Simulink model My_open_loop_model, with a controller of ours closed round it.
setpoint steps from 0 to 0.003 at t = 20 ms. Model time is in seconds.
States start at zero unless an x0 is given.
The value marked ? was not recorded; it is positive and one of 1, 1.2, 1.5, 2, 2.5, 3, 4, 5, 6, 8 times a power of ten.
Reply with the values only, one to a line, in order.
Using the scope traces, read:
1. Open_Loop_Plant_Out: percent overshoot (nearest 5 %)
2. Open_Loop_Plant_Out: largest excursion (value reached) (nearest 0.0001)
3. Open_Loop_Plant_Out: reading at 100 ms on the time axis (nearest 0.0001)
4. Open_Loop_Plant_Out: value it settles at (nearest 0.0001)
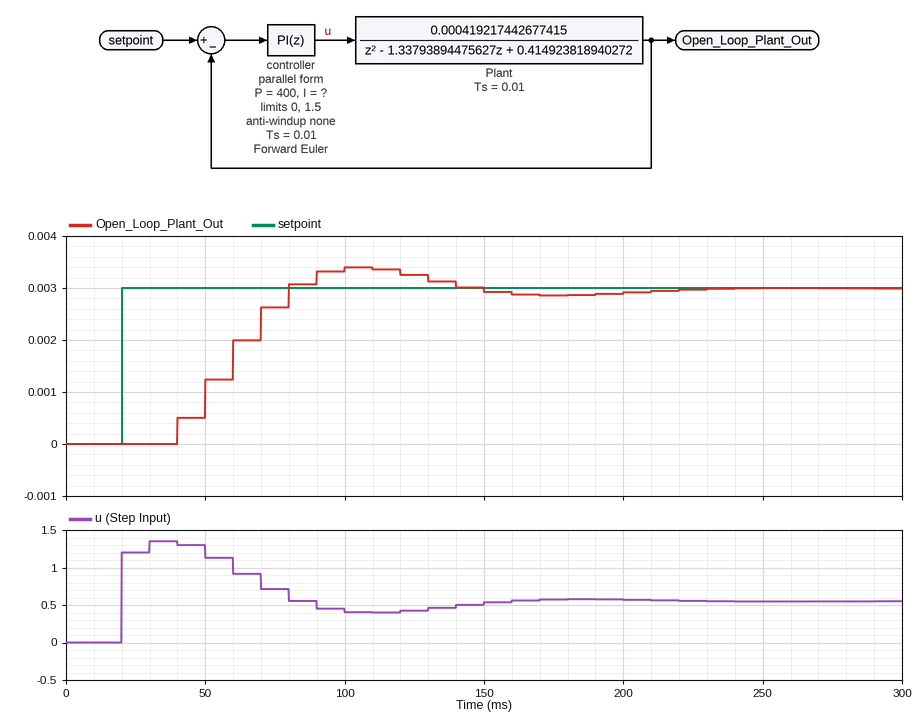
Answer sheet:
15 %
0.0034
0.0034
0.0030
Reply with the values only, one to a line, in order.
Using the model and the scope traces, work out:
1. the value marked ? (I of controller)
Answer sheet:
5000
